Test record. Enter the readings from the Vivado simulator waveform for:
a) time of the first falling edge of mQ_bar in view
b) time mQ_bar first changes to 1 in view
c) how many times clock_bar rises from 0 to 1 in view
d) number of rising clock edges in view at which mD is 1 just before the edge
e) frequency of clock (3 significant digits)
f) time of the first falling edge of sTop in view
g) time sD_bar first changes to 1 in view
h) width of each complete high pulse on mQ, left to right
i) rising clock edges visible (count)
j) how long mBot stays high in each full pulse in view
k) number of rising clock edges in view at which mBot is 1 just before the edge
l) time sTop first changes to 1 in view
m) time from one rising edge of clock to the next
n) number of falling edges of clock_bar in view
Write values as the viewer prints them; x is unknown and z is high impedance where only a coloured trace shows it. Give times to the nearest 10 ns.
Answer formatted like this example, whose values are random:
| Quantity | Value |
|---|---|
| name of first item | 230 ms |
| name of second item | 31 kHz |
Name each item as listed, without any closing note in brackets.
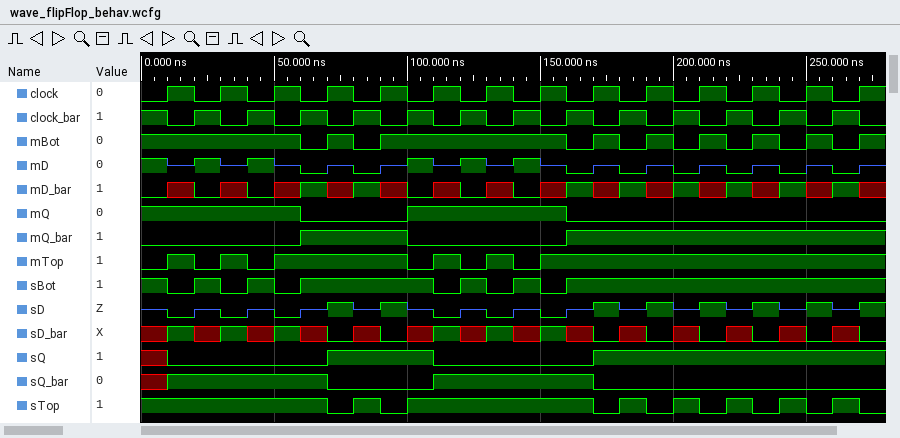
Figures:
| Quantity | Value |
|---|---|
| time of the first falling edge of mQ_bar in view | 100 ns |
| time mQ_bar first changes to 1 in view | 60 ns |
| how many times clock_bar rises from 0 to 1 in view | 13 |
| number of rising clock edges in view at which mD is 1 just before the edge | 6 |
| frequency of clock | 50.0 MHz |
| time of the first falling edge of sTop in view | 70 ns |
| time sD_bar first changes to 1 in view | 10 ns |
| width of each complete high pulse on mQ, left to right | 60 ns |
| rising clock edges visible | 14 |
| how long mBot stays high in each full pulse in view | 10 ns, 70 ns, 10 ns, 10 ns, 10 ns, 10 ns, 10 ns |
| number of rising clock edges in view at which mBot is 1 just before the edge | 6 |
| time sTop first changes to 1 in view | 80 ns |
| time from one rising edge of clock to the next | 20 ns |
| number of falling edges of clock_bar in view | 14 |
